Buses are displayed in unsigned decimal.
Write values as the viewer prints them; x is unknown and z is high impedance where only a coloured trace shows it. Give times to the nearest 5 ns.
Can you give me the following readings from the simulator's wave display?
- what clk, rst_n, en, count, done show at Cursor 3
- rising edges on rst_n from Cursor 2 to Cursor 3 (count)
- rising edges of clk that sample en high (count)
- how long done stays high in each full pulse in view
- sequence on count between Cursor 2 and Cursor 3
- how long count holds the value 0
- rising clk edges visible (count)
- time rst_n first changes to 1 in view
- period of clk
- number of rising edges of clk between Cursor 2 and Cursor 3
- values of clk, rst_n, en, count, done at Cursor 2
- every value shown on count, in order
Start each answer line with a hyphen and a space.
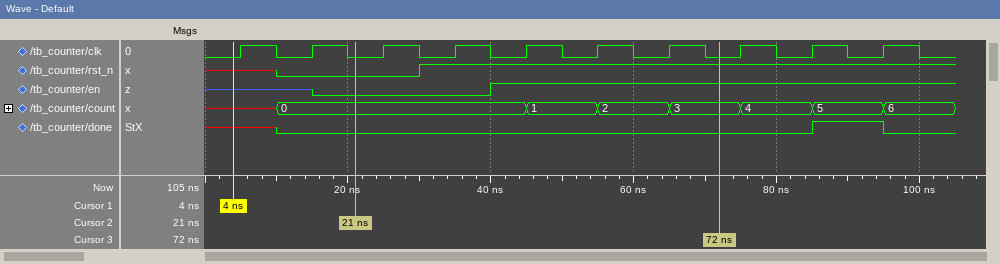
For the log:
- clk=0, rst_n=1, en=1, count=3, done=0
- 1
- 6
- 10 ns
- 0, 1, 2, 3
- 35 ns
- 10
- 30 ns
- 10 ns
- 5
- clk=0, rst_n=0, en=0, count=0, done=0
- x, 0, 1, 2, 3, 4, 5, 6
